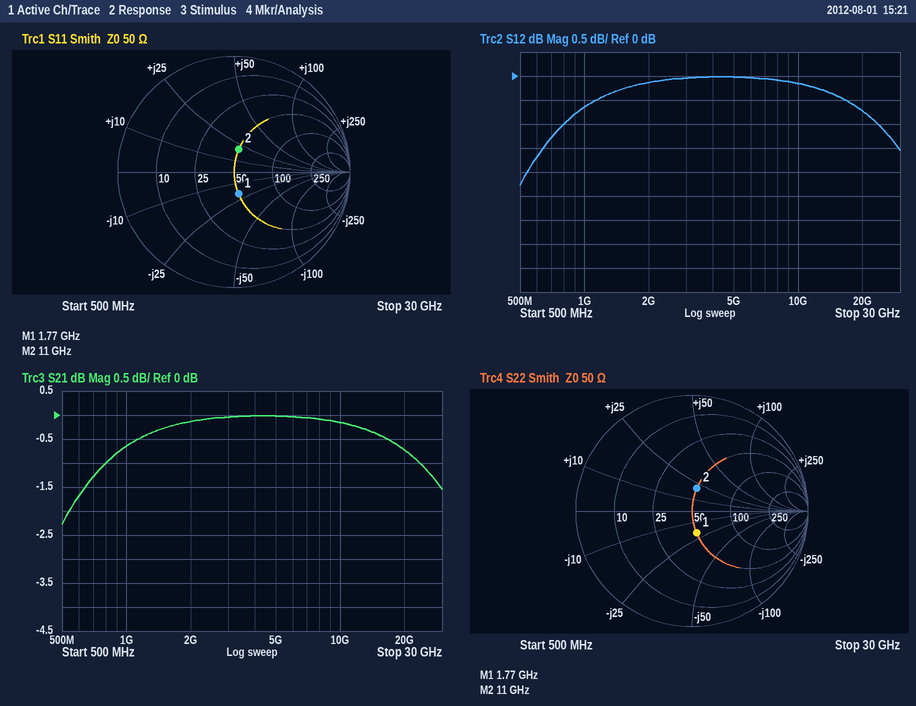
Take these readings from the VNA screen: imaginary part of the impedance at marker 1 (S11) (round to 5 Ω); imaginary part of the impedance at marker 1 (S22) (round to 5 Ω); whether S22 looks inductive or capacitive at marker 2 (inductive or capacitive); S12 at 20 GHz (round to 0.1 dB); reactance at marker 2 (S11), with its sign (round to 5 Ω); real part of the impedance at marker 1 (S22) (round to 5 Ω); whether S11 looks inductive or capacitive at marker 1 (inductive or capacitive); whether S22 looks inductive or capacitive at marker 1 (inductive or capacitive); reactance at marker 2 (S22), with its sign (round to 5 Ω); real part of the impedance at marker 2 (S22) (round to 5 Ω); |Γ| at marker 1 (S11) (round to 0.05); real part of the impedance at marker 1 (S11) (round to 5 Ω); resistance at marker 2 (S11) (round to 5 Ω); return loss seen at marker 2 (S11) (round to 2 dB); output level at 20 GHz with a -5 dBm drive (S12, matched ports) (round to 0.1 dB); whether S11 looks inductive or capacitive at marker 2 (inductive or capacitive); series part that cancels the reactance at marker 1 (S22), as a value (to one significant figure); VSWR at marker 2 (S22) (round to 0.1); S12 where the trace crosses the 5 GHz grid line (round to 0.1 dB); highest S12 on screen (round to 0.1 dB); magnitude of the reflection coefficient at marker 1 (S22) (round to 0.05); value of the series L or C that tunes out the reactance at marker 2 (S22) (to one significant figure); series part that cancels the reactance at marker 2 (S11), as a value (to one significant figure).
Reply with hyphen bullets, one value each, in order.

- -20 Ω
- -20 Ω
- inductive
- -0.7 dB
- +20 Ω
- 50 Ω
- capacitive
- capacitive
- +20 Ω
- 50 Ω
- 0.20
- 50 Ω
- 50 Ω
- 14 dB
- -5.7 dBm
- inductive
- 2 nH
- 1.5
- 0.0 dB
- 0.0 dB
- 0.20
- 700 fF
- 700 fF
